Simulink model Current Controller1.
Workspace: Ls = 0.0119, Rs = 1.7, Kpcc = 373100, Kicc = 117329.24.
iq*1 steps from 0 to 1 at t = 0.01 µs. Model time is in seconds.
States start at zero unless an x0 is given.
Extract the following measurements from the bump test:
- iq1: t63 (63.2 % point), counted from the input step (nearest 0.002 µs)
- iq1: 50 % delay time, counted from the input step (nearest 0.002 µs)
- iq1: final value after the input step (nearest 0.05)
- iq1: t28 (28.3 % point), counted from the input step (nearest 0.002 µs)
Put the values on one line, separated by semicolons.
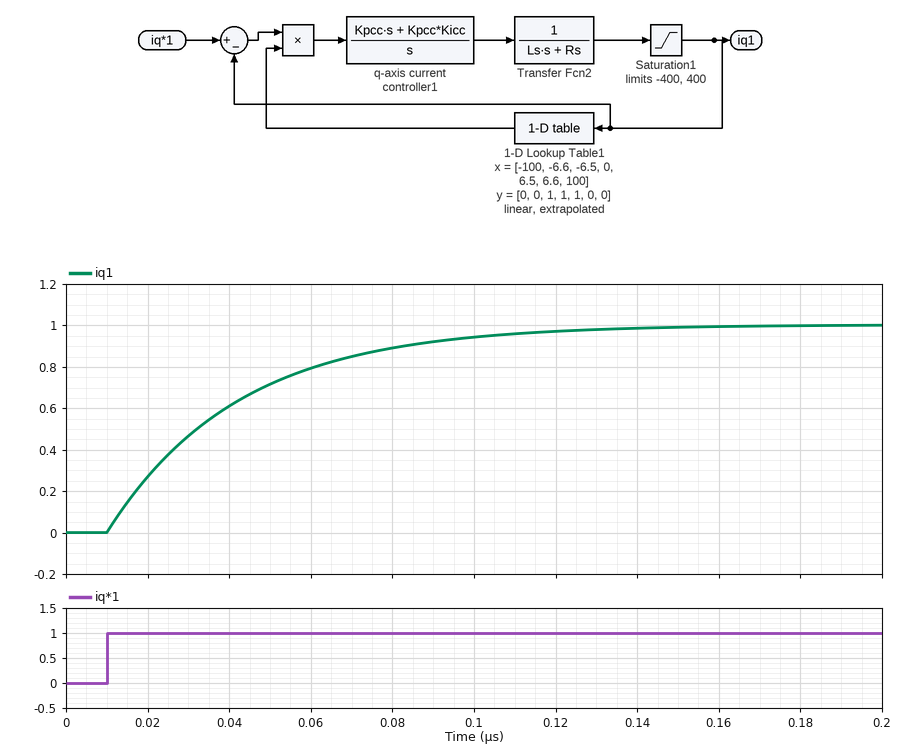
0.032 µs; 0.022 µs; 1.00; 0.010 µs
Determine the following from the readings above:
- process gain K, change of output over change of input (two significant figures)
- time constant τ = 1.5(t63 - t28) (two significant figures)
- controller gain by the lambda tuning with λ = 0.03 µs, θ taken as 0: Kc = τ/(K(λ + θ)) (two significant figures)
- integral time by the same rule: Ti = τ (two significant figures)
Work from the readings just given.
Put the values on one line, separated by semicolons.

1.0; 0.033 µs; 1.1; 0.033 µs
